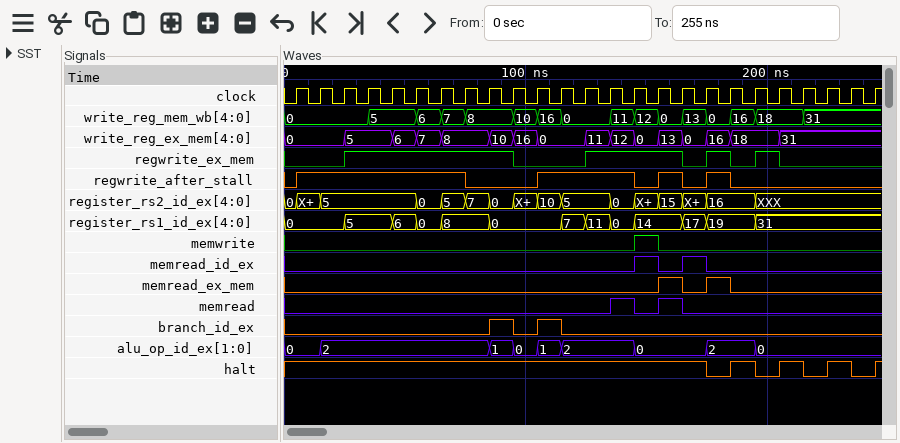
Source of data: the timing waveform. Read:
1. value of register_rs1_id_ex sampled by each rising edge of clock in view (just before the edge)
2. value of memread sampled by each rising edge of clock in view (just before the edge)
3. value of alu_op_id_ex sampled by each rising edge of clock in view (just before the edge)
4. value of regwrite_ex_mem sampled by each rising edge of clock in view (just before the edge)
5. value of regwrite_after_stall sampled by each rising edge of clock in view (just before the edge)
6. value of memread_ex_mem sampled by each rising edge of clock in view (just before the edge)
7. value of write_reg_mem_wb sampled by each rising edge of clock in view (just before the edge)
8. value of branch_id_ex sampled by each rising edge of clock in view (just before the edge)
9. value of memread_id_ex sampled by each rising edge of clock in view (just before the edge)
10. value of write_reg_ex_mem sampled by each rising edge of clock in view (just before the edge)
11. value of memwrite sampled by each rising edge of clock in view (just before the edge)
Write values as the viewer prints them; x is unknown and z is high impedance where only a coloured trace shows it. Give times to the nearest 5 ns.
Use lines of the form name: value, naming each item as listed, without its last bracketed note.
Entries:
value of register_rs1_id_ex sampled by each rising edge of clock in view: 0, 0, 0, 5, 5, 6, 0, 8, 8, 0, 0, 0, 7, 11, 0, 14, 14, 17, 19, 19, 31, 31, 31, 31, 31
value of memread sampled by each rising edge of clock in view: 0 0 0 0 0 0 0 0 0 0 0 0 0 0 1 0 1 0 0 0 0 0 0 0 0
value of alu_op_id_ex sampled by each rising edge of clock in view: 0, 0, 2, 2, 2, 2, 2, 2, 2, 1, 0, 1, 2, 2, 2, 0, 0, 0, 2, 2, 0, 0, 0, 0, 0
value of regwrite_ex_mem sampled by each rising edge of clock in view: 0 0 0 1 1 1 1 1 1 1 0 0 0 1 1 1 1 0 1 0 1 0 0 0 0
value of regwrite_after_stall sampled by each rising edge of clock in view: 0 1 1 1 1 1 1 1 0 0 0 1 1 1 1 0 1 0 1 0 0 0 0 0 0
value of memread_ex_mem sampled by each rising edge of clock in view: 0 0 0 0 0 0 0 0 0 0 0 0 0 0 0 0 1 0 1 0 0 0 0 0 0
value of write_reg_mem_wb sampled by each rising edge of clock in view: 0, 0, 0, 0, 5, 5, 6, 7, 8, 8, 10, 16, 0, 0, 11, 12, 0, 13, 0, 16, 18, 18, 31, 31, 31
value of branch_id_ex sampled by each rising edge of clock in view: 0 0 0 0 0 0 0 0 0 1 0 1 0 0 0 0 0 0 0 0 0 0 0 0 0
value of memread_id_ex sampled by each rising edge of clock in view: 0 0 0 0 0 0 0 0 0 0 0 0 0 0 0 1 0 1 0 0 0 0 0 0 0
value of write_reg_ex_mem sampled by each rising edge of clock in view: 0, 0, 0, 5, 5, 6, 7, 8, 8, 10, 16, 0, 0, 11, 12, 0, 13, 0, 16, 18, 18, 31, 31, 31, 31
value of memwrite sampled by each rising edge of clock in view: 0 0 0 0 0 0 0 0 0 0 0 0 0 0 0 1 0 0 0 0 0 0 0 0 0
